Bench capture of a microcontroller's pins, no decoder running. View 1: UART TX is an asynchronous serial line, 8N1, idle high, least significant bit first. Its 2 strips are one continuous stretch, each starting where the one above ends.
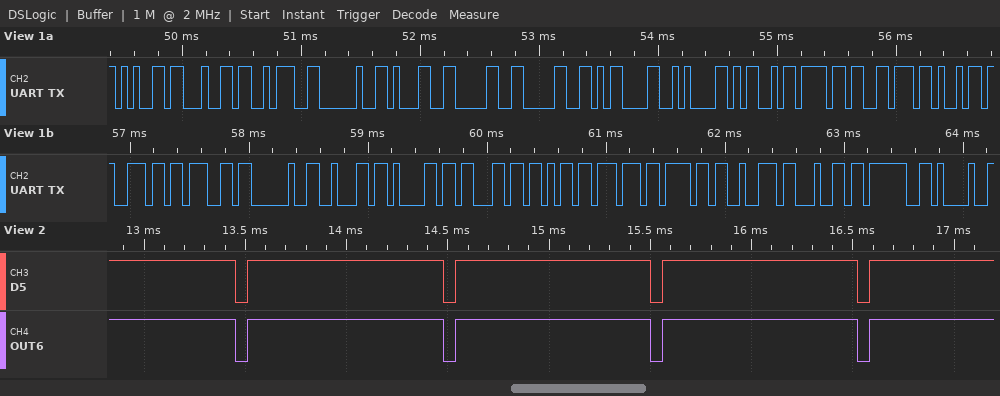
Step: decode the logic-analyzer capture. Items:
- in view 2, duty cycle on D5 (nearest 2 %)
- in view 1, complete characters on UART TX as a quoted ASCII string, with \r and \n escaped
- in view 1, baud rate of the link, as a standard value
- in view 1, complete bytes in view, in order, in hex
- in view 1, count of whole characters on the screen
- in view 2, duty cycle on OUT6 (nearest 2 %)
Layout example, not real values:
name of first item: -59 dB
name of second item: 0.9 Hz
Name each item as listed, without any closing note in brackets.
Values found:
in view 2, duty cycle on D5: 94 %
in view 1, complete characters on UART TX as a quoted ASCII string, with \r and \n escaped: "ed: 100\r\nMoving backword?!"
in view 1, baud rate of the link, as a standard value: 19200 baud
in view 1, complete bytes in view, in order, in hex: 65 64 3A 20 31 30 30 0D 0A 4D 6F 76 69 6E 67 20 62 61 63 6B 77 6F 72 64 3F 21
in view 1, count of whole characters on the screen: 26
in view 2, duty cycle on OUT6: 94 %
